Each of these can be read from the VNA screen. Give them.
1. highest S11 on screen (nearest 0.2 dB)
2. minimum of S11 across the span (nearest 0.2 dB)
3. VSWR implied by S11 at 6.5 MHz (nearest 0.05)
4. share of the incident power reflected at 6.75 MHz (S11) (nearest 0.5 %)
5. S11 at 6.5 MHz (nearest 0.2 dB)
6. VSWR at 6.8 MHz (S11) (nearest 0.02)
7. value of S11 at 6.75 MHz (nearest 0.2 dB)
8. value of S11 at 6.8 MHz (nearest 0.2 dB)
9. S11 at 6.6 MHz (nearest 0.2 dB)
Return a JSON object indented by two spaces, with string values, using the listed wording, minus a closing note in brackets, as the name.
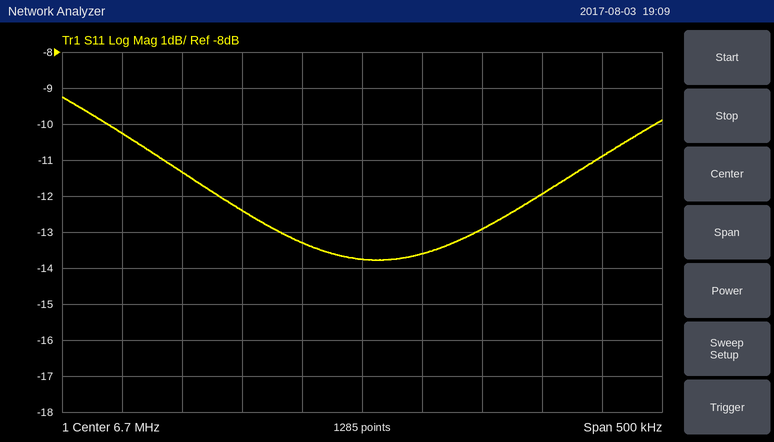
{
  "highest S11 on screen": "-9.2 dB",
  "minimum of S11 across the span": "-13.8 dB",
  "VSWR implied by S11 at 6.5 MHz": "1.90",
  "share of the incident power reflected at 6.75 MHz (S11)": "4.5 %",
  "S11 at 6.5 MHz": "-10.2 dB",
  "VSWR at 6.8 MHz (S11)": "1.58",
  "value of S11 at 6.75 MHz": "-13.6 dB",
  "value of S11 at 6.8 MHz": "-13.0 dB",
  "S11 at 6.6 MHz": "-12.4 dB"
}
